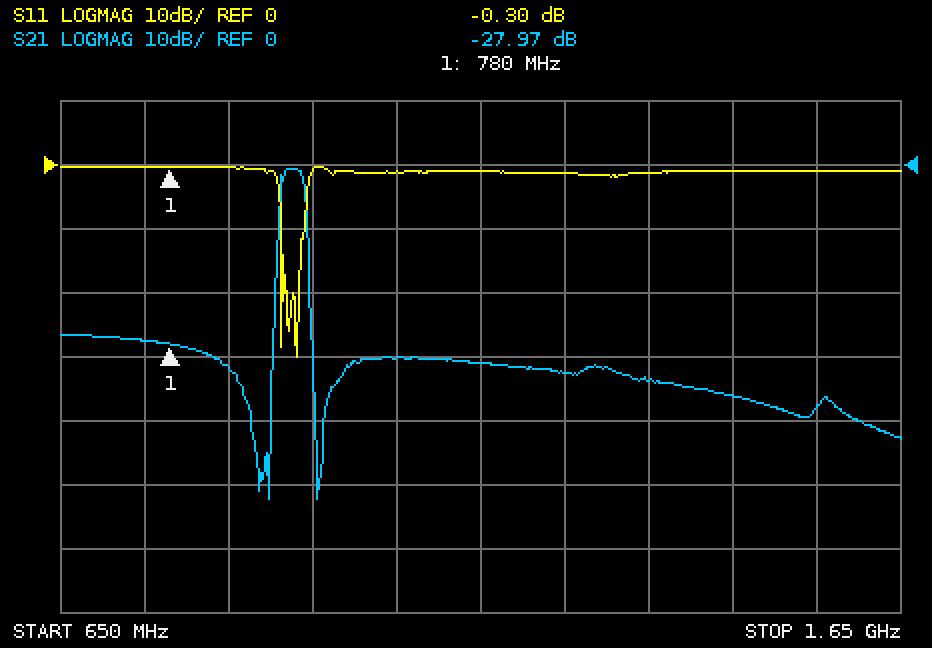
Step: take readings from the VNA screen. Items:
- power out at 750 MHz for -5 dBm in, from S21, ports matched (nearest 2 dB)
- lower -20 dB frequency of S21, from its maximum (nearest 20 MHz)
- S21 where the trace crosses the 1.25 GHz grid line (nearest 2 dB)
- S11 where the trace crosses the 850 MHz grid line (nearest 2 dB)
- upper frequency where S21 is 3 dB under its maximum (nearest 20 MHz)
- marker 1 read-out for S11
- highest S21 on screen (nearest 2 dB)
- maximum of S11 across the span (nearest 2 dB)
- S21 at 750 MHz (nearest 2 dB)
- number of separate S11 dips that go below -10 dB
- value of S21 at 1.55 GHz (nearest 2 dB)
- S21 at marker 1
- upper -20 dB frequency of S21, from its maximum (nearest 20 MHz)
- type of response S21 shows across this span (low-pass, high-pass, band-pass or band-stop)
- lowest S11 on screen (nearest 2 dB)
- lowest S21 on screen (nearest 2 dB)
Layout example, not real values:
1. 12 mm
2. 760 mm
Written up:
1. -32 dBm
2. 900 MHz
3. -32 dB
4. 0 dB
5. 940 MHz
6. -0.30 dB
7. 0 dB
8. 0 dB
9. -28 dB
10. 3
11. -38 dB
12. -27.97 dB
13. 940 MHz
14. band-pass
15. -30 dB
16. -52 dB
